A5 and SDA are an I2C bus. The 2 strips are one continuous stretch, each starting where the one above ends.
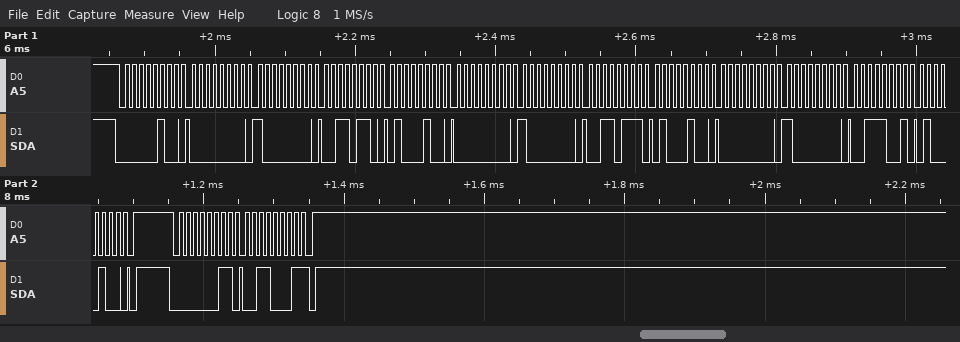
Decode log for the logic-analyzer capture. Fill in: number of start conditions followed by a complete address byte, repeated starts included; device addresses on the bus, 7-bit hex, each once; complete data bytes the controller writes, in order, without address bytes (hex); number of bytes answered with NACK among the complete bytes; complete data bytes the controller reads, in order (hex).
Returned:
2
0x02 0x01
00 80 36 44 00 80 37 44 00 80 39 44
1
31
